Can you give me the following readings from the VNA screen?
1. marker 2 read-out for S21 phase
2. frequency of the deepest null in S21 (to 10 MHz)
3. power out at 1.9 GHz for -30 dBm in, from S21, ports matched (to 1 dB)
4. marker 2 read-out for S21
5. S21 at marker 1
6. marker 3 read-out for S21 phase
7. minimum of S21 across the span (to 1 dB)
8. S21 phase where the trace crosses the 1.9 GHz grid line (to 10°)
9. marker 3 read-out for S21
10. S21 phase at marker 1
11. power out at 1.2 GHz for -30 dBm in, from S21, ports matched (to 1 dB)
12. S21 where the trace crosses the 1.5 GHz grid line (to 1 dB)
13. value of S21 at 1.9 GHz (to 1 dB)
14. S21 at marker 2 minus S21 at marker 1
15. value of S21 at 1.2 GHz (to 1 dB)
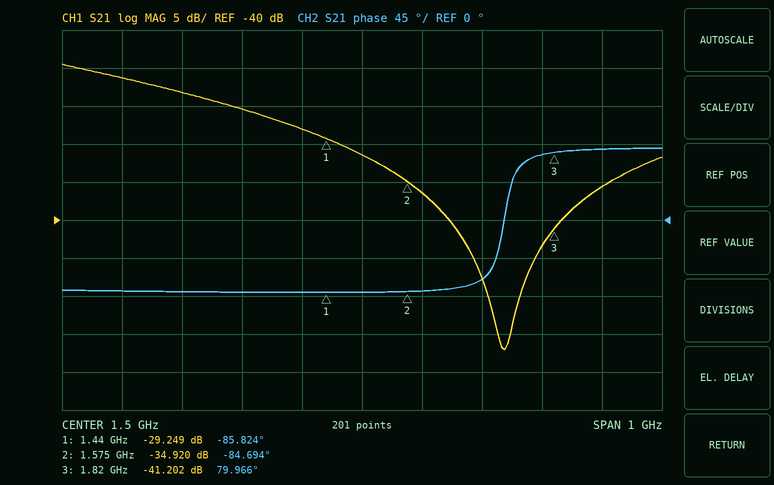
-84.694°
1.74 GHz
-66 dBm
-34.920 dB
-29.249 dB
79.966°
-57 dB
80°
-41.202 dB
-85.824°
-53 dBm
-31 dB
-36 dB
-5.671 dB
-23 dB
